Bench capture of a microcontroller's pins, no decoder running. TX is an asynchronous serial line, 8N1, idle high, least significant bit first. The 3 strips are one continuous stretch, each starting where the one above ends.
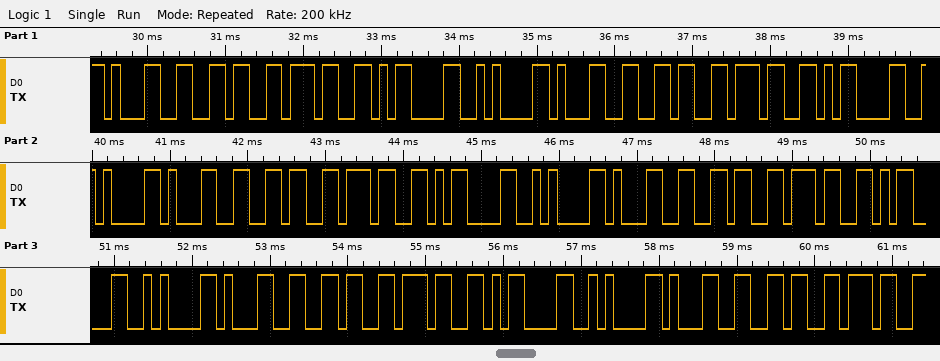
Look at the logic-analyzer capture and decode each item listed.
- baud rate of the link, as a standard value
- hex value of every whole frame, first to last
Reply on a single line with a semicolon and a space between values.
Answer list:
9600 baud; 31 36 37 0D 0A 31 36 37 0D 0A 31 36 37 0D 0A 31 36 37 0D 0A 31 36 37 0D 0A 31 36 37
